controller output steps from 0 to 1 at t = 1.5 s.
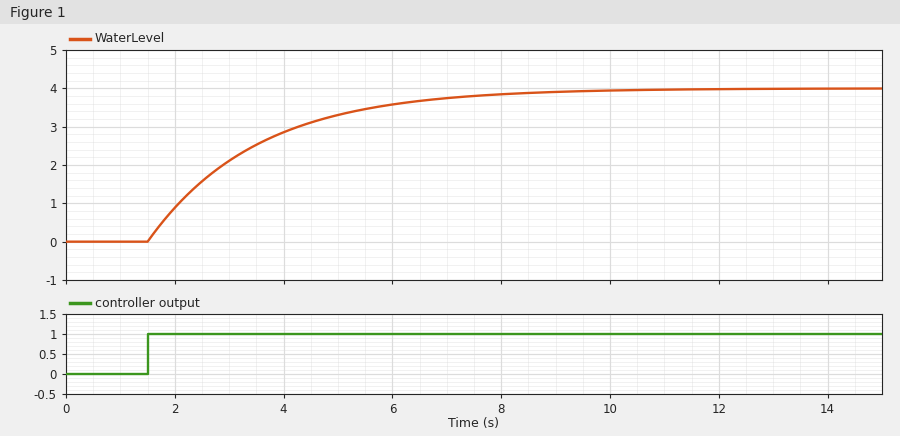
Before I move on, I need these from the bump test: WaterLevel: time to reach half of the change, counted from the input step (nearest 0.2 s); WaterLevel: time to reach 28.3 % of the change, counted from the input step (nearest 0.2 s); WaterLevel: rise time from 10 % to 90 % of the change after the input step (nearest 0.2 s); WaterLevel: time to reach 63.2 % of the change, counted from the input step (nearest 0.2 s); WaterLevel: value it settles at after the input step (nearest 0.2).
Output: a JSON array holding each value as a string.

["1.4 s", "0.6 s", "4.4 s", "2.0 s", "4.0"]
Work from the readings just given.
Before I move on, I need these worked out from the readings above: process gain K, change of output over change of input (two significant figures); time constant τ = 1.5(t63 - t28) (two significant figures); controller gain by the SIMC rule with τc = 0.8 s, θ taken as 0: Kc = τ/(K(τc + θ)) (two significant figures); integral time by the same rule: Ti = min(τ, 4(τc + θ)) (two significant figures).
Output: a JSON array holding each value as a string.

["4.0", "2.1 s", "0.66", "2.1 s"]
